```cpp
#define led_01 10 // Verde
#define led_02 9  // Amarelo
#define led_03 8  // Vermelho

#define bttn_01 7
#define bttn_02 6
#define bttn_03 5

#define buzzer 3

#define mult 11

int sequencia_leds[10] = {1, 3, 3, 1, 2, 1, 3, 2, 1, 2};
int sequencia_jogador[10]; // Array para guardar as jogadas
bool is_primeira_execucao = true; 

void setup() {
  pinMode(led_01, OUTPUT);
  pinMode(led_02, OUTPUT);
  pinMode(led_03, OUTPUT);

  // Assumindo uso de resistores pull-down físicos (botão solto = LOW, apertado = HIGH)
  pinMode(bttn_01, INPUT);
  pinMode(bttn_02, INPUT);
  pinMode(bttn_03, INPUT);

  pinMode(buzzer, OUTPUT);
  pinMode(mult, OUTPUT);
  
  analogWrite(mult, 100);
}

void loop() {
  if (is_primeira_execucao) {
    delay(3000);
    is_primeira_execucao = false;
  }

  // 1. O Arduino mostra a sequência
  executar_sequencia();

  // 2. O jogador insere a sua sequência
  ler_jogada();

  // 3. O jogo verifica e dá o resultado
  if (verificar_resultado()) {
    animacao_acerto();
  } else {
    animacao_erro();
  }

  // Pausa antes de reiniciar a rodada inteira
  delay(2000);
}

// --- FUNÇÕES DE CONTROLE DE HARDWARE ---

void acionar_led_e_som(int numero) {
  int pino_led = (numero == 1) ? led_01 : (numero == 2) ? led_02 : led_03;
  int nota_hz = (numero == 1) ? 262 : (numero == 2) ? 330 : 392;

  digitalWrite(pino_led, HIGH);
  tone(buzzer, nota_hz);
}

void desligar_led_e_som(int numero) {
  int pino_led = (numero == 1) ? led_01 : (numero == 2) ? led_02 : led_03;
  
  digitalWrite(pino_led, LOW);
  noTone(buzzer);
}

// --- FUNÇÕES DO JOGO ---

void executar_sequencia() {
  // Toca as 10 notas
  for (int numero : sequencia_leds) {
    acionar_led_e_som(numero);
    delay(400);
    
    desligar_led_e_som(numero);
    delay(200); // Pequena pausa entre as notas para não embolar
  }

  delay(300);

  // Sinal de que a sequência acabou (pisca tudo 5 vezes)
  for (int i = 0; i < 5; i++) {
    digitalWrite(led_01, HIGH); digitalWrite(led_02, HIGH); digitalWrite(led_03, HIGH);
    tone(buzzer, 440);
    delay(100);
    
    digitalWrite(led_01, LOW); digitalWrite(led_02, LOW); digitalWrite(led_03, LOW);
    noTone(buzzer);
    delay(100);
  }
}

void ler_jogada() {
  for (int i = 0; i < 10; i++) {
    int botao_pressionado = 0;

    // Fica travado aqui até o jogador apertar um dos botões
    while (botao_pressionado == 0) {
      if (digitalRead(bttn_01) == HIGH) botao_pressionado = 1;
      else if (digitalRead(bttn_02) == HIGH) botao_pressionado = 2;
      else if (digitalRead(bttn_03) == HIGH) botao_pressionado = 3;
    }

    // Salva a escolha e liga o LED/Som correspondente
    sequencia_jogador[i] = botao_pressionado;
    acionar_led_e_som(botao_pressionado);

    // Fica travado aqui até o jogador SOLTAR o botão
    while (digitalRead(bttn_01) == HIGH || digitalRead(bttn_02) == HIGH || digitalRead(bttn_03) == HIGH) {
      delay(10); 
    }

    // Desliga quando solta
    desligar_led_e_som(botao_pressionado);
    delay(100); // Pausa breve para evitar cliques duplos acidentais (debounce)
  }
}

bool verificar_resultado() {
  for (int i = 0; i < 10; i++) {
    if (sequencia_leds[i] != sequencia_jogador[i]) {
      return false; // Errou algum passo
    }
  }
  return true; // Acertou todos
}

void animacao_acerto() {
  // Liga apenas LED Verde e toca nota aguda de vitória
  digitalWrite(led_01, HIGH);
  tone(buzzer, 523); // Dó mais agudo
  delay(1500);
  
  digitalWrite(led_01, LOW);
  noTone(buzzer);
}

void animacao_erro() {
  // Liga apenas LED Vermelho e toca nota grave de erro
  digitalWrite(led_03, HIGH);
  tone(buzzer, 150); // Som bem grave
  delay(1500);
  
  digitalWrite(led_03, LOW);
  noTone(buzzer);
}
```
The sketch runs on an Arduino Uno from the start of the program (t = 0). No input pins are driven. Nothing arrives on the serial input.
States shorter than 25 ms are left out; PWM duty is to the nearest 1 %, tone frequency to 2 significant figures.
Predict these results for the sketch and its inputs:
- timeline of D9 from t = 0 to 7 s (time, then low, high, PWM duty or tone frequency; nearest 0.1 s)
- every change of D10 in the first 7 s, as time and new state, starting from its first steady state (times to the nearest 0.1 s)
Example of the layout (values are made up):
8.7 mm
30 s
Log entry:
0 s low; 5.4 s high; 5.8 s low
0 s low; 3 s high; 3.4 s low; 4.8 s high; 5.2 s low; 6 s high; 6.4 s low
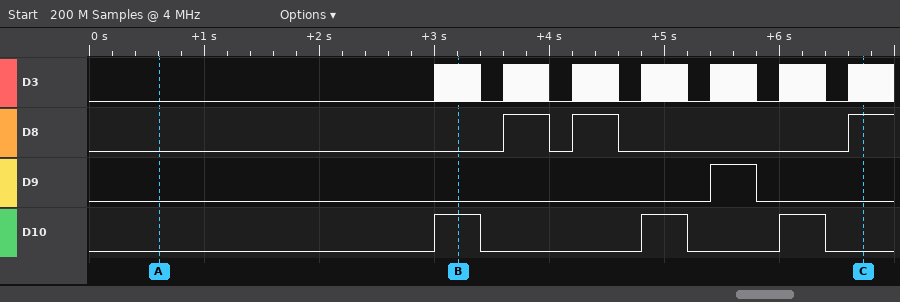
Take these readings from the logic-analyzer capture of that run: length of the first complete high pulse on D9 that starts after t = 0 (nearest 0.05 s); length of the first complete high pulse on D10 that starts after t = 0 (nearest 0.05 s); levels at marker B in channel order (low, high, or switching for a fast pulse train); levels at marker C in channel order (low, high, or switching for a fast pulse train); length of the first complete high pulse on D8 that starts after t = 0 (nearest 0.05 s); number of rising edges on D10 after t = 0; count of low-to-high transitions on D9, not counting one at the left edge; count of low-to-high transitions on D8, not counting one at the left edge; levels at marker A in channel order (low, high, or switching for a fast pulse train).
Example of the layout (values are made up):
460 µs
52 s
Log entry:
0.40 s
0.40 s
D3 switching, D8 low, D9 low, D10 high
D3 switching, D8 high, D9 low, D10 low
0.40 s
3
1
3
D3 low, D8 low, D9 low, D10 low
